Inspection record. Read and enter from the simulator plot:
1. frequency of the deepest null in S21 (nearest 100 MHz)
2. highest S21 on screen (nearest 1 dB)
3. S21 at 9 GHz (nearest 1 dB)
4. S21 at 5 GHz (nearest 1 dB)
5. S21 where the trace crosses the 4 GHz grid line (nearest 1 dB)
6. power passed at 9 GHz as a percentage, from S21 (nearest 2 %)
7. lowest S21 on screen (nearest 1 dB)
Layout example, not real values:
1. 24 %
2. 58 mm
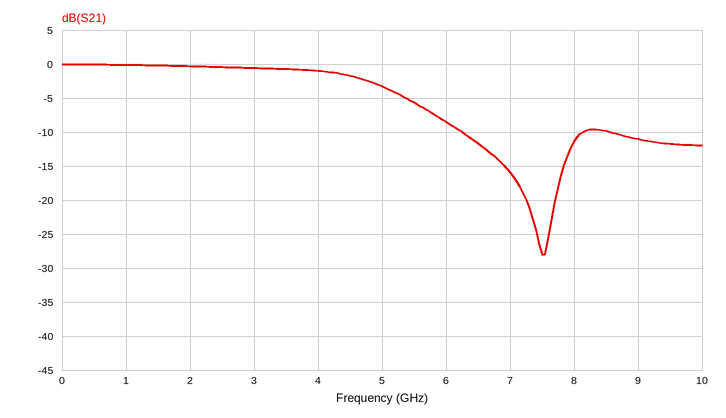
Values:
1. 7.5 GHz
2. 0 dB
3. -11 dB
4. -3 dB
5. -1 dB
6. 8 %
7. -28 dB
